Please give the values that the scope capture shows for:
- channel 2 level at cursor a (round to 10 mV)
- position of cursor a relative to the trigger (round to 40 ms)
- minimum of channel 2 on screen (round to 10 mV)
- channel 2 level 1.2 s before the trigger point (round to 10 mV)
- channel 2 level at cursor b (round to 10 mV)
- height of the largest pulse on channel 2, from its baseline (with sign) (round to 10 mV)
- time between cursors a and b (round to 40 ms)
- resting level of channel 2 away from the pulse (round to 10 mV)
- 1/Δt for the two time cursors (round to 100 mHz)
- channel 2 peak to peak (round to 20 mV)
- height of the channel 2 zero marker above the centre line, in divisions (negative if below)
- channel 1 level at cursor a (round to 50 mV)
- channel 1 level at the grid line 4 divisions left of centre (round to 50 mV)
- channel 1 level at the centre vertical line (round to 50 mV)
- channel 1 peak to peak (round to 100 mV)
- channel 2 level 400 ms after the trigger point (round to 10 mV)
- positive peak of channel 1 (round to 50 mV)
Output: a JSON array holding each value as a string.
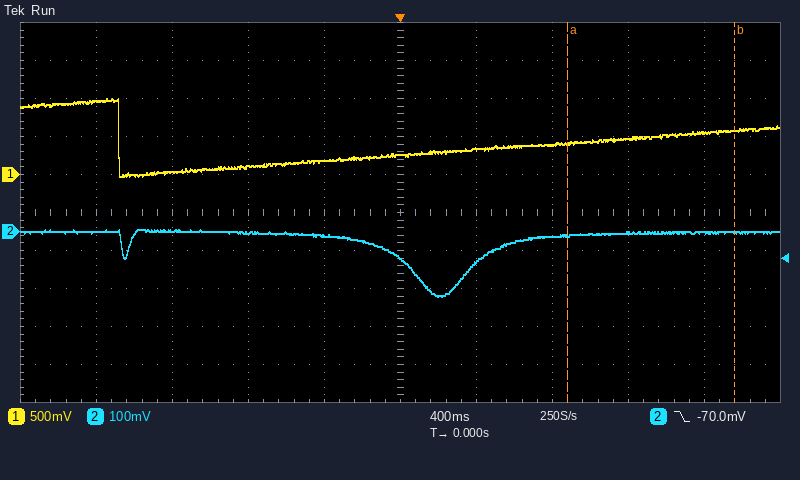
["-10 mV", "+880 ms", "-170 mV", "0 mV", "0 mV", "-170 mV", "880 ms", "0 mV", "1.1 Hz", "180 mV", "-0.5 div", "400 mV", "950 mV", "250 mV", "1.00 V", "-80 mV", "1.00 V"]
